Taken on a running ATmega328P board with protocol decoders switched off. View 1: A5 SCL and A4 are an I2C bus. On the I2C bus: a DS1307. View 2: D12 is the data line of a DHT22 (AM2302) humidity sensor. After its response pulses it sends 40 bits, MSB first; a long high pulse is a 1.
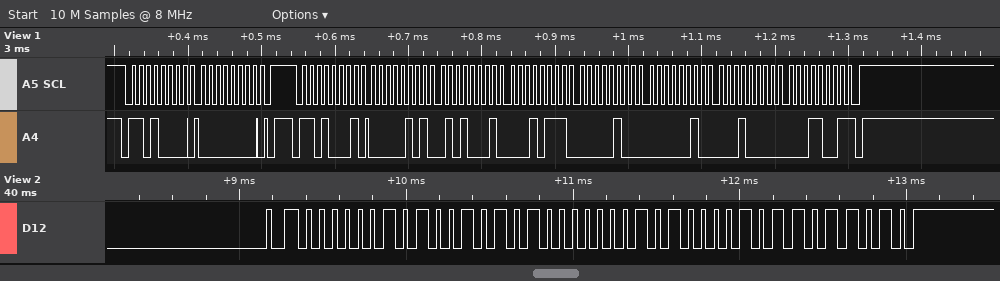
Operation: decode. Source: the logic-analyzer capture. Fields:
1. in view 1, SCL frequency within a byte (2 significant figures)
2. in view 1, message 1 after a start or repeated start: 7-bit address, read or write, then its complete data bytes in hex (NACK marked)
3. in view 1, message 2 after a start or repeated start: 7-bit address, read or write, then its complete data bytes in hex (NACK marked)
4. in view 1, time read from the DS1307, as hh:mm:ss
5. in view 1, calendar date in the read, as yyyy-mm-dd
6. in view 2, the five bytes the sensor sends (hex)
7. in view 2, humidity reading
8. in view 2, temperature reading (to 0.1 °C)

100 kHz
0x68 write: 00
0x68 read: 05 51 17 04 02 10 19 NACK
17:51:05
2019-10-02
02 95 01 42 DA
66.1 %
32.2 °C
